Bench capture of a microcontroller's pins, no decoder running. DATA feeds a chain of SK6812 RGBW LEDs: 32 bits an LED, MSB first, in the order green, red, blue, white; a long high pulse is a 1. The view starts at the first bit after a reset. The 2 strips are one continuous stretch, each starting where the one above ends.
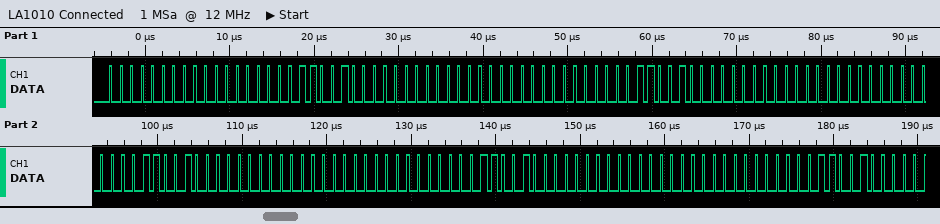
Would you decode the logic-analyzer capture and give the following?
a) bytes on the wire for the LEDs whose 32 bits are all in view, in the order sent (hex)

00 00 32 00 00 00 32 00 00 00 32 00 00 00 32 00
